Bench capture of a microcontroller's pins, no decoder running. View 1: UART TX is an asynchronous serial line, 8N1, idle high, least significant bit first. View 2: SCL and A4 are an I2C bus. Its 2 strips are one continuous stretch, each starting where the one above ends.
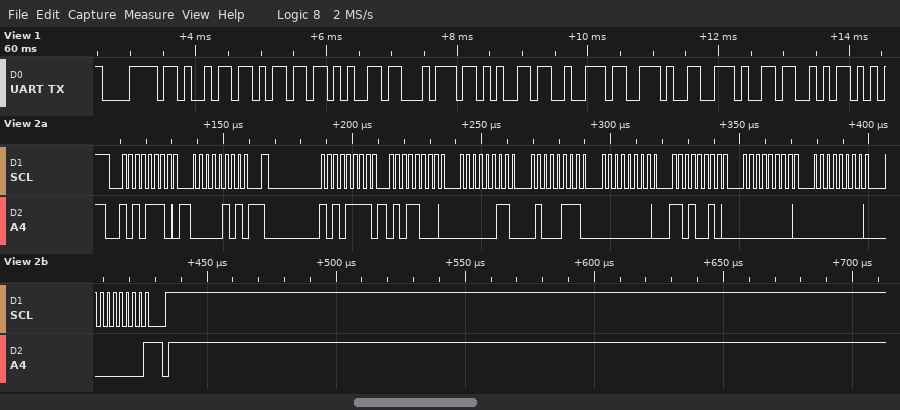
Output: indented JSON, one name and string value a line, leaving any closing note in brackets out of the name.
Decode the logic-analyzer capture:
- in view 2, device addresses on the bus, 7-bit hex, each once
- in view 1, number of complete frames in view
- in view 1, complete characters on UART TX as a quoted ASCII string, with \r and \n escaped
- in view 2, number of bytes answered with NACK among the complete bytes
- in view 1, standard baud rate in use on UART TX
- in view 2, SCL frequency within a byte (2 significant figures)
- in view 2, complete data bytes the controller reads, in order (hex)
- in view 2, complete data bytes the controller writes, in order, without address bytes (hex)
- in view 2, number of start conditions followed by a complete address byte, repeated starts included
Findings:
{
  "in view 2, device addresses on the bus, 7-bit hex, each once": "0x57",
  "in view 1, number of complete frames in view": "10",
  "in view 1, complete characters on UART TX as a quoted ASCII string, with \\r and \\n escaped": "\"ximeter..S\"",
  "in view 2, number of bytes answered with NACK among the complete bytes": "1",
  "in view 1, standard baud rate in use on UART TX": "9600 baud",
  "in view 2, SCL frequency within a byte": "400 kHz",
  "in view 2, complete data bytes the controller reads, in order": "58 03 47 00 D2 00 00 00",
  "in view 2, complete data bytes the controller writes, in order, without address bytes": "05",
  "in view 2, number of start conditions followed by a complete address byte, repeated starts included": "2"
}
